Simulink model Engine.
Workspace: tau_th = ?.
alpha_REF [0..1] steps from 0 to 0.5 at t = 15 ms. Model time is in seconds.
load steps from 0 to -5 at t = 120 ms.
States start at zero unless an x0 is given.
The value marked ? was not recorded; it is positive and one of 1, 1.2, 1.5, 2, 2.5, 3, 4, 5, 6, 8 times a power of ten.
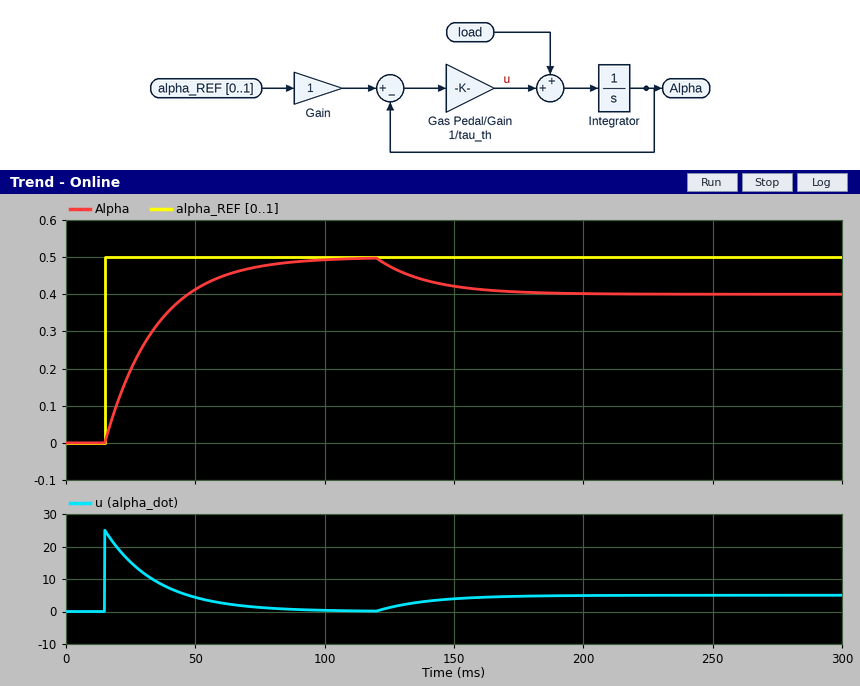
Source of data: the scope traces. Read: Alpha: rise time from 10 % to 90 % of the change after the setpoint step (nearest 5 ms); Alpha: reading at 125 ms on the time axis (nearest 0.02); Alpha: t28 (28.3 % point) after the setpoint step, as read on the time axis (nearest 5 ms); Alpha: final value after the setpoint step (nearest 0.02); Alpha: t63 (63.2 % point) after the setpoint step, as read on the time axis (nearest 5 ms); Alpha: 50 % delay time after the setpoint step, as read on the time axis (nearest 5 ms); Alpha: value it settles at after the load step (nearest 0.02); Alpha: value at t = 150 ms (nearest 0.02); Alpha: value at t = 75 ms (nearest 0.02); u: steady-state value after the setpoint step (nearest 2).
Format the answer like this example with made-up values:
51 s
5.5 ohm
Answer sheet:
45 ms
0.48
20 ms
0.50
35 ms
30 ms
0.40
0.42
0.48
0
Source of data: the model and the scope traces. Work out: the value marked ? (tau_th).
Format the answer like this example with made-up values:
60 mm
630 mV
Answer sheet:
0.02
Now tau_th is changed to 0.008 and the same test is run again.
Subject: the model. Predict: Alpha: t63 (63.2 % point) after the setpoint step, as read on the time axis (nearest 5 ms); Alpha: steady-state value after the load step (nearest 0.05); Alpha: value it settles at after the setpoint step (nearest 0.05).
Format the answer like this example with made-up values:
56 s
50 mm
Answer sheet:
25 ms
0.45
0.50
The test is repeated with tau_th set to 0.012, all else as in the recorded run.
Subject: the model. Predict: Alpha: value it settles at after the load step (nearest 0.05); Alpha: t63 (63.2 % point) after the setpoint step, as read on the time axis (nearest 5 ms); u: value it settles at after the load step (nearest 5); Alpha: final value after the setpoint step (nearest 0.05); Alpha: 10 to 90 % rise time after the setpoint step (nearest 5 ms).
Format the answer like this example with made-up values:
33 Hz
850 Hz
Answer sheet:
0.45
25 ms
5
0.50
25 ms
